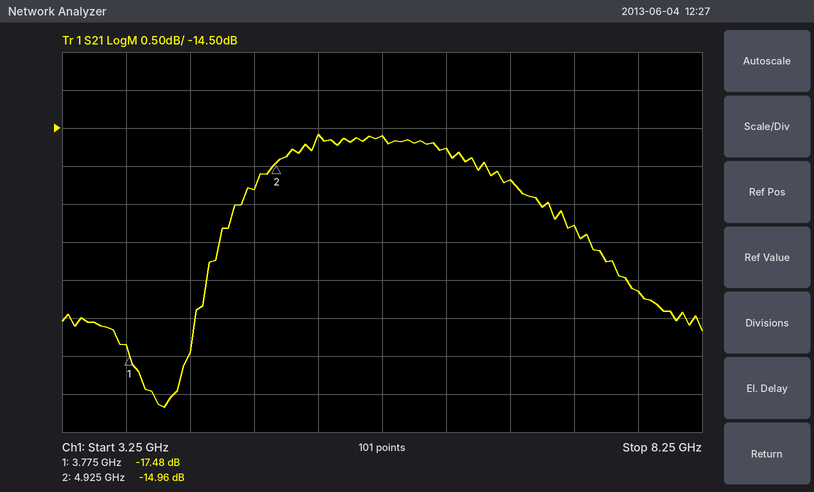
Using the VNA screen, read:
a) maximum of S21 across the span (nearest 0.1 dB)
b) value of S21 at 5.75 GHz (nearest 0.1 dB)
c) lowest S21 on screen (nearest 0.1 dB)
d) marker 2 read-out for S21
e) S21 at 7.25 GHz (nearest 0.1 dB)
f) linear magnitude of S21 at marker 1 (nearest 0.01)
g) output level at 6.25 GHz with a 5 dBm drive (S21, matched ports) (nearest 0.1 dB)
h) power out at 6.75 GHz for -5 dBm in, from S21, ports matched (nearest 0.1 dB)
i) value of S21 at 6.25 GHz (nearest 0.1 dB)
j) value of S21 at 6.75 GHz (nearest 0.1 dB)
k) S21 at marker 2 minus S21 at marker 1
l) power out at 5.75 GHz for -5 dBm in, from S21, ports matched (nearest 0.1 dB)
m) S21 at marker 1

-14.6 dB
-14.6 dB
-18.2 dB
-14.96 dB
-15.8 dB
0.13
-9.8 dBm
-20.2 dBm
-14.8 dB
-15.2 dB
2.52 dB
-19.6 dBm
-17.48 dB
